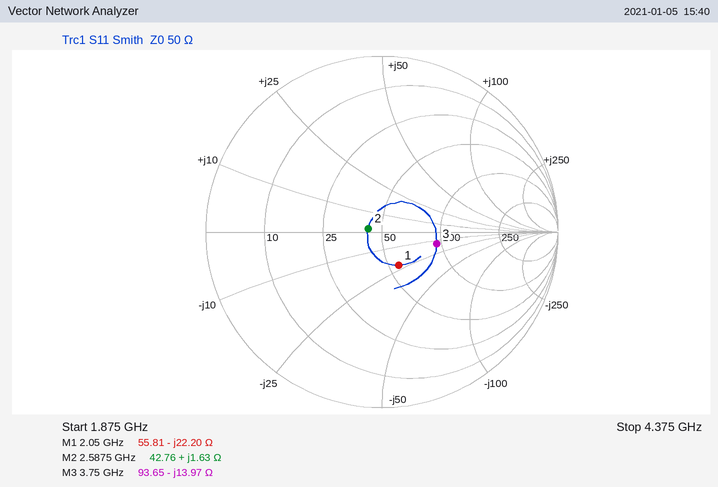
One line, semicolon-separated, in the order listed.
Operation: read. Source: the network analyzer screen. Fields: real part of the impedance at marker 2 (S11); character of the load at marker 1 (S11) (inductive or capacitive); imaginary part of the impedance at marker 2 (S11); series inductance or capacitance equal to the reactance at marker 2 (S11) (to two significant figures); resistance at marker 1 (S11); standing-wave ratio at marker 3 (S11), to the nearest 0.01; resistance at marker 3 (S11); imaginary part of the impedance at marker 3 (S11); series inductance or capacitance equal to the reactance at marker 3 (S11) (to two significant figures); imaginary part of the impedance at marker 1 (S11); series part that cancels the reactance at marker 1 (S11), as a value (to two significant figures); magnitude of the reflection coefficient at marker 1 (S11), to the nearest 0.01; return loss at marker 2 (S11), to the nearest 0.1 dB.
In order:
42.76 Ω; capacitive; +1.63 Ω; 100 pH; 55.81 Ω; 1.93; 93.65 Ω; -13.97 Ω; 3.0 pF; -22.20 Ω; 1.7 nH; 0.21; 21.9 dB
